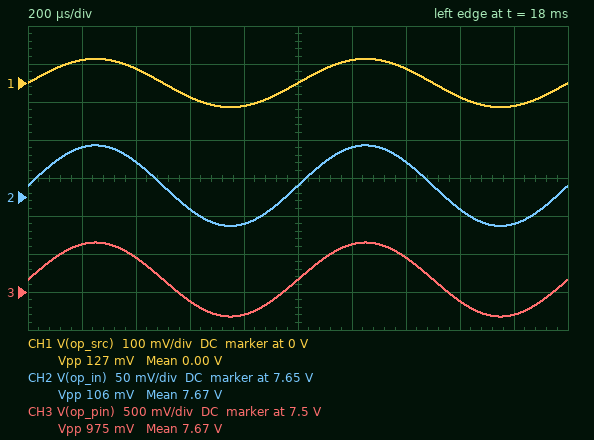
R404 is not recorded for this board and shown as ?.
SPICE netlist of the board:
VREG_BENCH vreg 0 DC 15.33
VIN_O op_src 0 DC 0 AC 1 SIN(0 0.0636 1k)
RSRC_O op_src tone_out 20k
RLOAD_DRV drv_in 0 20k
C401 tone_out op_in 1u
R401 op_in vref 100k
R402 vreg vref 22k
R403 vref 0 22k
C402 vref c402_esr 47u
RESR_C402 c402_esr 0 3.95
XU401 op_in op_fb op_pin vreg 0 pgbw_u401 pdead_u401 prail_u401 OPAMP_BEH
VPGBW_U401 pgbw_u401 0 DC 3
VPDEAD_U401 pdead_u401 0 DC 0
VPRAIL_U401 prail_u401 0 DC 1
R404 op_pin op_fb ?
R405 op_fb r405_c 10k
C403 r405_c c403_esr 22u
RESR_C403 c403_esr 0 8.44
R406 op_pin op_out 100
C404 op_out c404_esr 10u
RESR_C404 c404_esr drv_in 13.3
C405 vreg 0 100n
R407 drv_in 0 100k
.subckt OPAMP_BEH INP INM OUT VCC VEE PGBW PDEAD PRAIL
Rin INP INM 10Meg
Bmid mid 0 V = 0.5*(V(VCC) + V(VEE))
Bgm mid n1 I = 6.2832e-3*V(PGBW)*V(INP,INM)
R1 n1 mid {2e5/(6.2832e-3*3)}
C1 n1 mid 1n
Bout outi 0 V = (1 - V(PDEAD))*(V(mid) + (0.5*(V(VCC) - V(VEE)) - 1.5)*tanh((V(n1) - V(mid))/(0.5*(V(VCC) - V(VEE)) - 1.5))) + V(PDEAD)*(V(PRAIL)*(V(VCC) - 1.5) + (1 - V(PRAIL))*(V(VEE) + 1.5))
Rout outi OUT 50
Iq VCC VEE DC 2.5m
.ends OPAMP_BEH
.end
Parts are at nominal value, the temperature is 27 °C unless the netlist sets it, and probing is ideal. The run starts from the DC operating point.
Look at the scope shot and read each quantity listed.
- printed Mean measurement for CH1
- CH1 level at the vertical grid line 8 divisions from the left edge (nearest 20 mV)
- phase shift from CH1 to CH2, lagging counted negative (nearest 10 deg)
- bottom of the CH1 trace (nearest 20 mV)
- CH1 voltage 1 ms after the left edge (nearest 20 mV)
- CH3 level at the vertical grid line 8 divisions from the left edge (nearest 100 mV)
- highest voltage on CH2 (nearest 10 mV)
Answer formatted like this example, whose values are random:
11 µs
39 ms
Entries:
0.00 V
-40 mV
0 deg
-60 mV
0 V
7.4 V
7.72 V
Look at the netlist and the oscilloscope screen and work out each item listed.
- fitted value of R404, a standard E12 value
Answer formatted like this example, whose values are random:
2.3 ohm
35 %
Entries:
82 kΩ
